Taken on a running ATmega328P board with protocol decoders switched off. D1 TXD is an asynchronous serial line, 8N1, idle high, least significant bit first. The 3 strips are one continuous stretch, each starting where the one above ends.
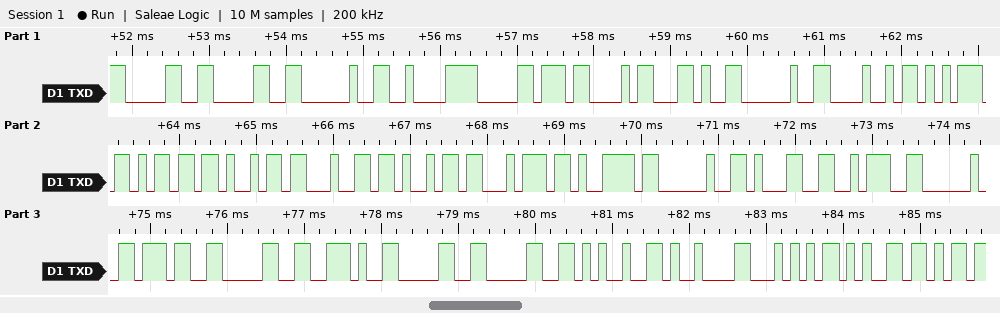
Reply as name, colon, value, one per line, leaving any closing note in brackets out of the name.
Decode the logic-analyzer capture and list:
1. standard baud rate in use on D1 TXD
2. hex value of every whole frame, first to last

standard baud rate in use on D1 TXD: 9600 baud
hex value of every whole frame, first to last: 0x30 0x30 0x20 0xC2 0xB0 0x43 0x2C 0x20 0x48 0x75 0x6D 0x69 0x64 0x69 0x74 0x79 0x20 0x31 0x3A 0x20 0x37 0x30 0x2E 0x30 0x30 0x25 0x09 0x54 0x65
